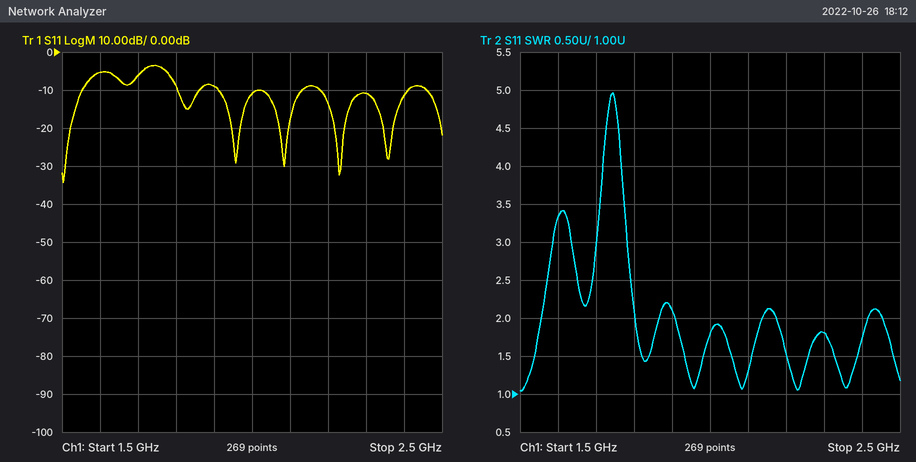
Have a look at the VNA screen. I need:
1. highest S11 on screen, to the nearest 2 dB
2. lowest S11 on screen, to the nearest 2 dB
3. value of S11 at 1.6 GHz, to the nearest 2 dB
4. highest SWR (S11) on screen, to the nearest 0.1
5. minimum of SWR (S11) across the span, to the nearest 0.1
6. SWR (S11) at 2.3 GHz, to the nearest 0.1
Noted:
-4 dB
-34 dB
-6 dB
5.0
1.0
1.8
